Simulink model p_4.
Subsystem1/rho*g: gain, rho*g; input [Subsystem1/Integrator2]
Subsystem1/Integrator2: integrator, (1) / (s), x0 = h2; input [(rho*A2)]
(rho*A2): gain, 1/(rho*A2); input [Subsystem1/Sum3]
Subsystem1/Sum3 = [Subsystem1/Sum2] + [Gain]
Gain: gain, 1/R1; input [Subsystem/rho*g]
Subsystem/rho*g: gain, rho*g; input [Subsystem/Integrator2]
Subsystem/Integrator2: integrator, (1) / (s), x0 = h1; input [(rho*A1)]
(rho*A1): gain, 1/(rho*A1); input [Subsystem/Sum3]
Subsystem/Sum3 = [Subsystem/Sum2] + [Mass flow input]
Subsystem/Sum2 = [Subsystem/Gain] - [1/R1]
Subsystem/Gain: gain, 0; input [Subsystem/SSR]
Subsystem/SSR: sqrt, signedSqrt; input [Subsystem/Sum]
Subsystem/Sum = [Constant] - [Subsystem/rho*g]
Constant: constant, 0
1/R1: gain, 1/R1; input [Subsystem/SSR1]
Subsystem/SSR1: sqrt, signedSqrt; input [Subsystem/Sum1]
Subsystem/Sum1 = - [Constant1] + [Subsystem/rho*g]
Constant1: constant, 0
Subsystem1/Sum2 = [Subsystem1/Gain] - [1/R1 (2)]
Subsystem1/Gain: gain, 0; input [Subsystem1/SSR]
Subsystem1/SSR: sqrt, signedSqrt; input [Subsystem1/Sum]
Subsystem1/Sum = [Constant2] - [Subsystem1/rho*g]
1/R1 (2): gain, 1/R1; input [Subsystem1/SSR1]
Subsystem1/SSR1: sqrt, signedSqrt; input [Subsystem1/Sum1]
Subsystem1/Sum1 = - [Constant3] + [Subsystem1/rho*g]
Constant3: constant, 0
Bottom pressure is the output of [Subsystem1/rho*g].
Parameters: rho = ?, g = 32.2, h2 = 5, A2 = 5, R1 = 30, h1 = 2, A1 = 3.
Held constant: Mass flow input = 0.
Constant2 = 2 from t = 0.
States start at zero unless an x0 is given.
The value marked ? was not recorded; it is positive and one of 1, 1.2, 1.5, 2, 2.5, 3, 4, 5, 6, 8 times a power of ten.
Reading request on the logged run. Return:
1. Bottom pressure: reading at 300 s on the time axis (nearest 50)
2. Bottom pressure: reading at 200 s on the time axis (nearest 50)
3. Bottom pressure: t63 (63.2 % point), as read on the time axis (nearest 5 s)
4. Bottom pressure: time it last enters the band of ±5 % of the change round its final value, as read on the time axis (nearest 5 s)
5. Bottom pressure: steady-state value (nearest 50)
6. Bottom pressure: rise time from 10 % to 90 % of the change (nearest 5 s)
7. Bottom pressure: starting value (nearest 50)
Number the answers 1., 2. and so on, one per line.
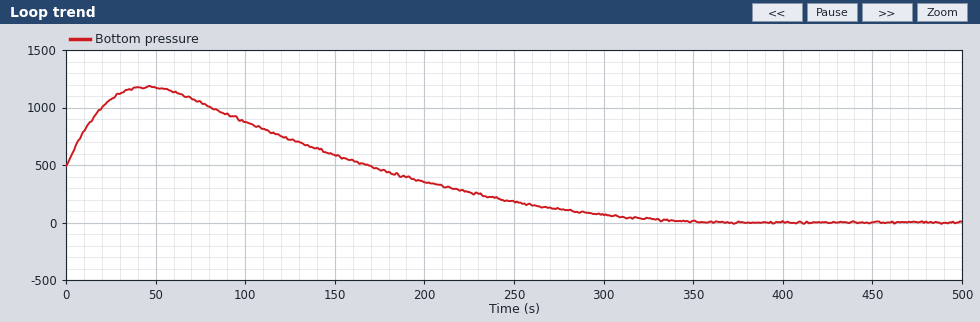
1. 50
2. 350
3. 250 s
4. 330 s
5. 0
6. 130 s
7. 500
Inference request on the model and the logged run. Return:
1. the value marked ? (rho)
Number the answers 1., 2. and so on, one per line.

1. 3
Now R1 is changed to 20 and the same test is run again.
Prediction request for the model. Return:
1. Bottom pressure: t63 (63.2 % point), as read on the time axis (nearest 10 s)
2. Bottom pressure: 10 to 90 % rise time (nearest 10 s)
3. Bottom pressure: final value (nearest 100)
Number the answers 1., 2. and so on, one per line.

1. 170 s
2. 90 s
3. 0
